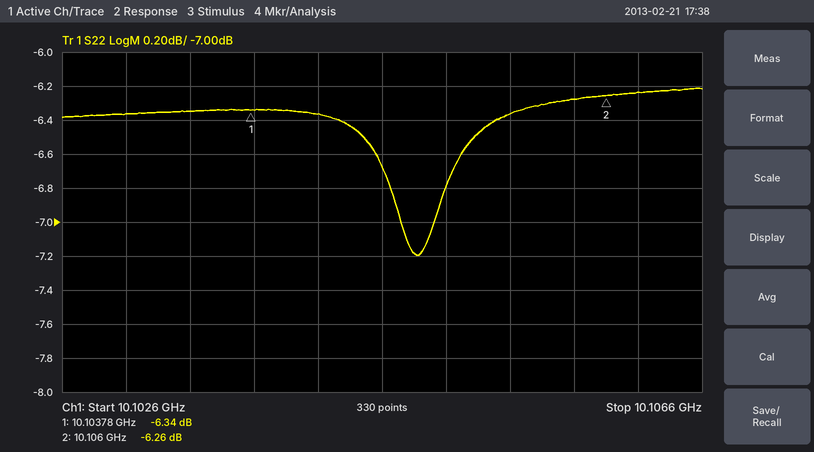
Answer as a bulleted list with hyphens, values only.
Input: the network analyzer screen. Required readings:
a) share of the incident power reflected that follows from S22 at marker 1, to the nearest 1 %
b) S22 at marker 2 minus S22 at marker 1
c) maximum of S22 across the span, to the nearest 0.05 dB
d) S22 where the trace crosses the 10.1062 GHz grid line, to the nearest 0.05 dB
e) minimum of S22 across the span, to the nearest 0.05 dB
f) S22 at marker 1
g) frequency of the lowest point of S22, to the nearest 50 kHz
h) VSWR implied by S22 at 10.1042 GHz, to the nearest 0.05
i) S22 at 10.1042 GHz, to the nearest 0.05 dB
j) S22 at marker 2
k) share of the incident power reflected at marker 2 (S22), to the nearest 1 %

- 23 %
- 0.08 dB
- -6.20 dB
- -6.25 dB
- -7.20 dB
- -6.34 dB
- 10.10480 GHz
- 2.85
- -6.35 dB
- -6.26 dB
- 24 %
